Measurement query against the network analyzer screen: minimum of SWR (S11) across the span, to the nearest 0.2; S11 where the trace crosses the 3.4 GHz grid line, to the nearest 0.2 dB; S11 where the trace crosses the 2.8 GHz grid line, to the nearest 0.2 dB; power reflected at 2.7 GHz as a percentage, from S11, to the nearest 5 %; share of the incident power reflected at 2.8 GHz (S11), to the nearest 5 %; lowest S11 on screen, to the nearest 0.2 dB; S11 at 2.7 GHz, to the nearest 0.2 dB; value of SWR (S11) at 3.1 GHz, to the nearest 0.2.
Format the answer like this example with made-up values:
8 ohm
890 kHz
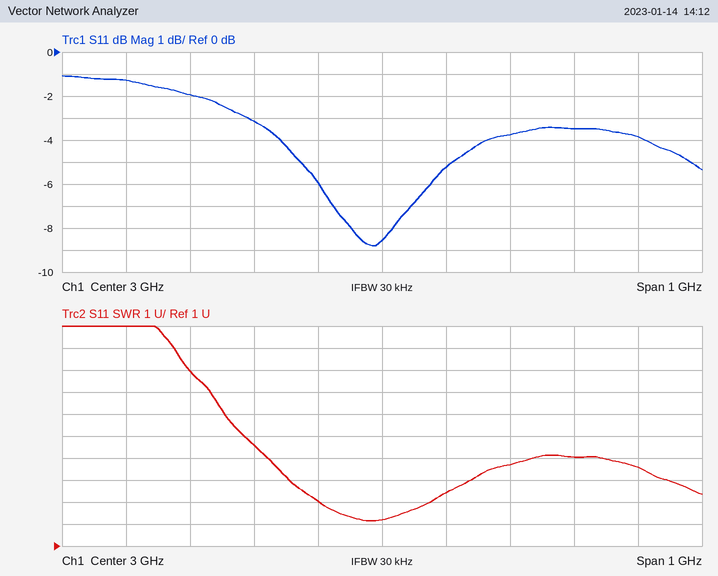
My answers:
2.2
-3.8 dB
-3.2 dB
65 %
50 %
-8.8 dB
-2.0 dB
3.4
